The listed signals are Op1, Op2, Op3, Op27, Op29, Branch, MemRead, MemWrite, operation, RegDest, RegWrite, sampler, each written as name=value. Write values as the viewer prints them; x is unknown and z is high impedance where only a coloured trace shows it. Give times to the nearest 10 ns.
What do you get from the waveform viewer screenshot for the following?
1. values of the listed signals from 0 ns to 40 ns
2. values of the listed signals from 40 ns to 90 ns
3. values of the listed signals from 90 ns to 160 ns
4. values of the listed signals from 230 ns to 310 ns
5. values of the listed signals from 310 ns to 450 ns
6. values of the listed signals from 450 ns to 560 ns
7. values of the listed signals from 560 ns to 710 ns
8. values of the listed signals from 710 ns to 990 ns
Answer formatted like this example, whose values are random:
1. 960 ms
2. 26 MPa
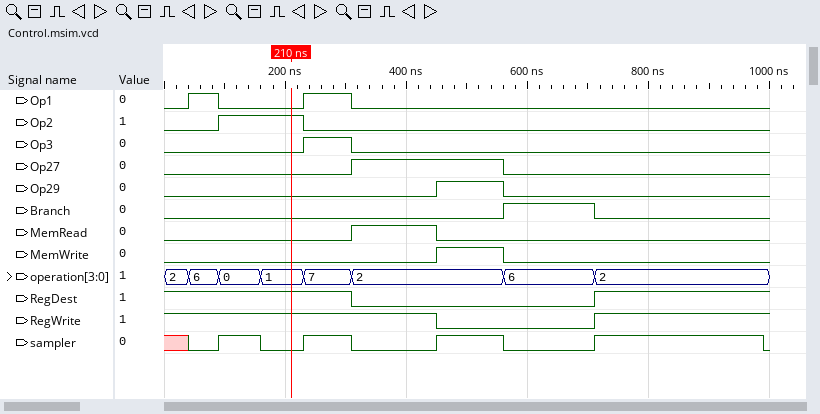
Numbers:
1. Op1=0, Op2=0, Op3=0, Op27=0, Op29=0, Branch=0, MemRead=0, MemWrite=0, operation=2, RegDest=1, RegWrite=1, sampler=x
2. Op1=1, Op2=0, Op3=0, Op27=0, Op29=0, Branch=0, MemRead=0, MemWrite=0, operation=6, RegDest=1, RegWrite=1, sampler=0
3. Op1=0, Op2=1, Op3=0, Op27=0, Op29=0, Branch=0, MemRead=0, MemWrite=0, operation=0, RegDest=1, RegWrite=1, sampler=1
4. Op1=1, Op2=0, Op3=1, Op27=0, Op29=0, Branch=0, MemRead=0, MemWrite=0, operation=7, RegDest=1, RegWrite=1, sampler=1
5. Op1=0, Op2=0, Op3=0, Op27=1, Op29=0, Branch=0, MemRead=1, MemWrite=0, operation=2, RegDest=0, RegWrite=1, sampler=0
6. Op1=0, Op2=0, Op3=0, Op27=1, Op29=1, Branch=0, MemRead=0, MemWrite=1, operation=2, RegDest=0, RegWrite=0, sampler=1
7. Op1=0, Op2=0, Op3=0, Op27=0, Op29=0, Branch=1, MemRead=0, MemWrite=0, operation=6, RegDest=0, RegWrite=0, sampler=0
8. Op1=0, Op2=0, Op3=0, Op27=0, Op29=0, Branch=0, MemRead=0, MemWrite=0, operation=2, RegDest=1, RegWrite=1, sampler=1
